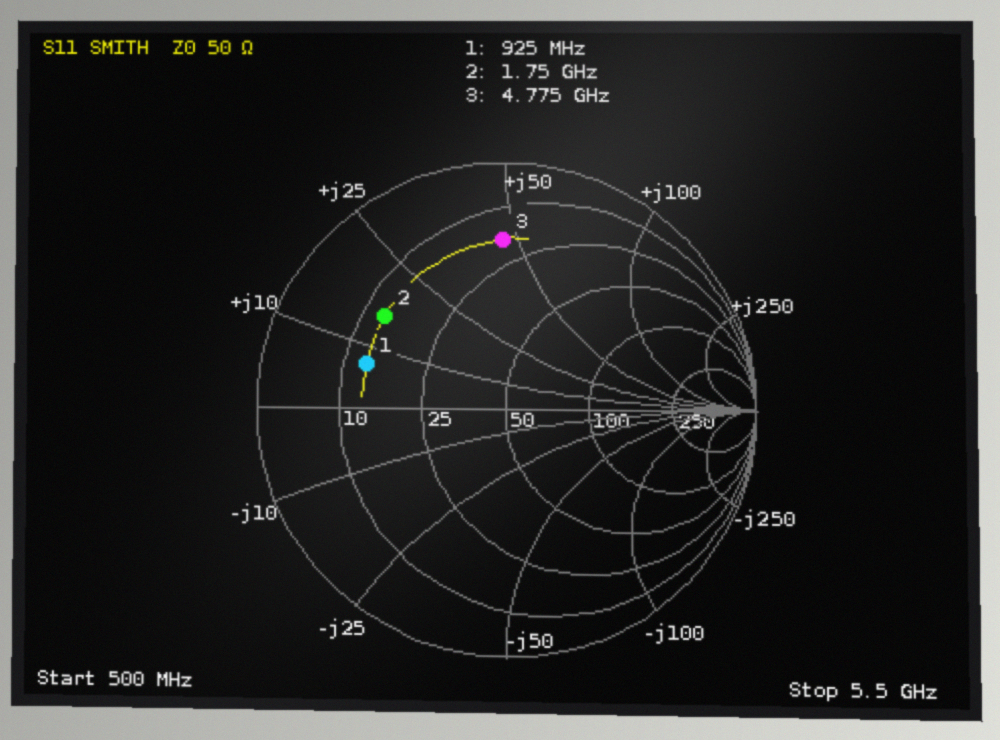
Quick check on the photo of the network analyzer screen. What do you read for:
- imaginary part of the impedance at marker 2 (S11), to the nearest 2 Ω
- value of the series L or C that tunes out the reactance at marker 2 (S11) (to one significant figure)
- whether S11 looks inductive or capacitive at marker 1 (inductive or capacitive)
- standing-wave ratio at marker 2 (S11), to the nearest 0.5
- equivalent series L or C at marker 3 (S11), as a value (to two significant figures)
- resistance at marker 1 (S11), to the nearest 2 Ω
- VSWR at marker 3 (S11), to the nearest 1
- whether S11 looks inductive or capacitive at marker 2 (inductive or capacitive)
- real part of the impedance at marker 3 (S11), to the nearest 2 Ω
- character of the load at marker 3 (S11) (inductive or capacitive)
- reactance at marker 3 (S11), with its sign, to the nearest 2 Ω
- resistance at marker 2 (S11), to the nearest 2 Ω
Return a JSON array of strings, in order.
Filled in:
["+16 Ω", "6 pF", "inductive", "4.0", "1.5 nH", "14 Ω", "5", "inductive", "18 Ω", "inductive", "+46 Ω", "14 Ω"]
